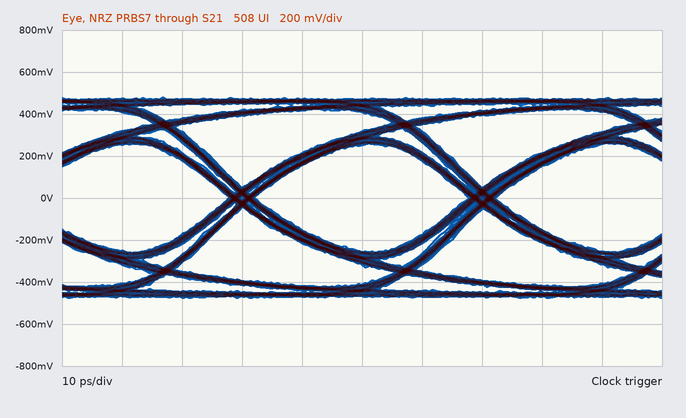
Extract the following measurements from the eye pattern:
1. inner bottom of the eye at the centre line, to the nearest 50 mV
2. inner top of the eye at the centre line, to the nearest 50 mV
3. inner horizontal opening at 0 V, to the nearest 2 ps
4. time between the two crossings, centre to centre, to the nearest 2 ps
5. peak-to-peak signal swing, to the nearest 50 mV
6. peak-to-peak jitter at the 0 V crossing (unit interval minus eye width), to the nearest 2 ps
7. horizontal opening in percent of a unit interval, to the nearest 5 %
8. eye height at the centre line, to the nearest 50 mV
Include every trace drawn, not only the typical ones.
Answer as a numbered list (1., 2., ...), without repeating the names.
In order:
1. -250 mV
2. 250 mV
3. 36 ps
4. 40 ps
5. 950 mV
6. 4 ps
7. 90 %
8. 500 mV
